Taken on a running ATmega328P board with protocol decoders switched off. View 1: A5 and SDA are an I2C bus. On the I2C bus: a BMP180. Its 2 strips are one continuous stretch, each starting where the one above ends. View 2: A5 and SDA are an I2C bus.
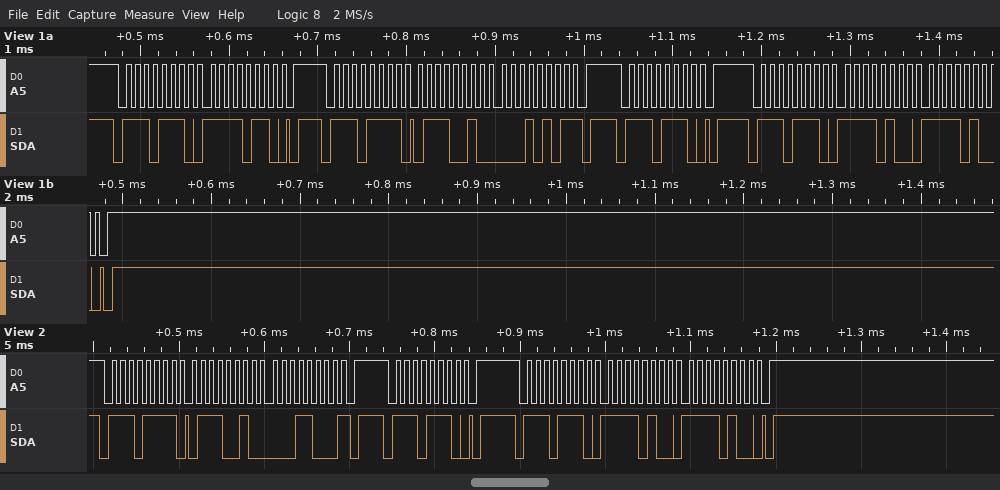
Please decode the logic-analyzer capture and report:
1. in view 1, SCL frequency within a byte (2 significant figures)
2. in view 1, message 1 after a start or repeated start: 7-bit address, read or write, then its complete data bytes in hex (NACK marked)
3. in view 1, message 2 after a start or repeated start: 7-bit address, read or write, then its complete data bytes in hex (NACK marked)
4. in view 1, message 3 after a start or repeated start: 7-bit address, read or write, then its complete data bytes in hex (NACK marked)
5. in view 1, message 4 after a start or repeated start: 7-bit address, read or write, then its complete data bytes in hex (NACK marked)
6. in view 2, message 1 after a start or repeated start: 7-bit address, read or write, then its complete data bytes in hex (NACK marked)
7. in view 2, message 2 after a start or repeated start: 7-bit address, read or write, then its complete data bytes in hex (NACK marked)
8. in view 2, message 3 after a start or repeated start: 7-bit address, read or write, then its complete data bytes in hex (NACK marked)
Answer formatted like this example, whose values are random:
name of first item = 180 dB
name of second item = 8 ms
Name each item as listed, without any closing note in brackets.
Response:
in view 1, SCL frequency within a byte = 100 kHz
in view 1, message 1 after a start or repeated start: 7-bit address, read or write, then its complete data bytes in hex = 0x77 write: F6
in view 1, message 2 after a start or repeated start: 7-bit address, read or write, then its complete data bytes in hex = 0x77 read: 72 15 NACK
in view 1, message 3 after a start or repeated start: 7-bit address, read or write, then its complete data bytes in hex = 0x77 write
in view 1, message 4 after a start or repeated start: 7-bit address, read or write, then its complete data bytes in hex = 0x77 write: F4 F4
in view 2, message 1 after a start or repeated start: 7-bit address, read or write, then its complete data bytes in hex = 0x77 read: 72 18 NACK
in view 2, message 2 after a start or repeated start: 7-bit address, read or write, then its complete data bytes in hex = 0x77 write
in view 2, message 3 after a start or repeated start: 7-bit address, read or write, then its complete data bytes in hex = 0x77 write: F4 F4
